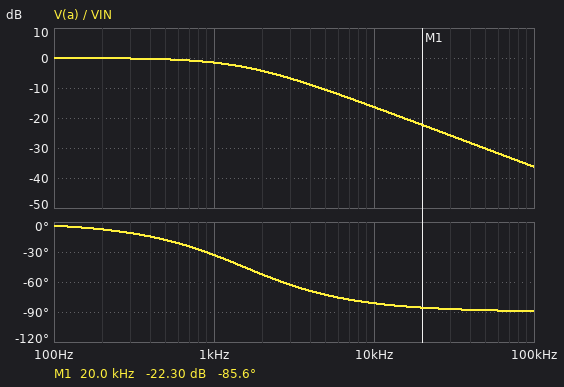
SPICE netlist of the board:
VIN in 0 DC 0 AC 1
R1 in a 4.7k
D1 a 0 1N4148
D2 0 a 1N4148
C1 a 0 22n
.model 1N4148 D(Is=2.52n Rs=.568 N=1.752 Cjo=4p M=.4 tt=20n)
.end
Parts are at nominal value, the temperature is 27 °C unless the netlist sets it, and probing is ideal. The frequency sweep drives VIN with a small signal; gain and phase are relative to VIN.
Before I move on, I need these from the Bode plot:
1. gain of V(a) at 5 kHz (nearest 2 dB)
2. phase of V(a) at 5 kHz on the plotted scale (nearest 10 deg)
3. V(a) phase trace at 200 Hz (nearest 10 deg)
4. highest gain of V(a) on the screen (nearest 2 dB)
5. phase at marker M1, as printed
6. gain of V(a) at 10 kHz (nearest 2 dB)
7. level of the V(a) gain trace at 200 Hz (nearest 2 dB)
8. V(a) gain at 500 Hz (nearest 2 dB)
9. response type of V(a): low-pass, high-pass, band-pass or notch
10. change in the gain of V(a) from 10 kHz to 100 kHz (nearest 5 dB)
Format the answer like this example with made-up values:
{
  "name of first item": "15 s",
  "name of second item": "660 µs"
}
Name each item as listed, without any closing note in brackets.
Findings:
{
  "gain of V(a) at 5 kHz": "-10 dB",
  "phase of V(a) at 5 kHz on the plotted scale": "-70 deg",
  "V(a) phase trace at 200 Hz": "-10 deg",
  "highest gain of V(a) on the screen": "0 dB",
  "phase at marker M1, as printed": "-85.6 deg",
  "gain of V(a) at 10 kHz": "-16 dB",
  "level of the V(a) gain trace at 200 Hz": "0 dB",
  "V(a) gain at 500 Hz": "0 dB",
  "response type of V(a): low-pass, high-pass, band-pass or notch": "low-pass",
  "change in the gain of V(a) from 10 kHz to 100 kHz": "-20 dB"
}
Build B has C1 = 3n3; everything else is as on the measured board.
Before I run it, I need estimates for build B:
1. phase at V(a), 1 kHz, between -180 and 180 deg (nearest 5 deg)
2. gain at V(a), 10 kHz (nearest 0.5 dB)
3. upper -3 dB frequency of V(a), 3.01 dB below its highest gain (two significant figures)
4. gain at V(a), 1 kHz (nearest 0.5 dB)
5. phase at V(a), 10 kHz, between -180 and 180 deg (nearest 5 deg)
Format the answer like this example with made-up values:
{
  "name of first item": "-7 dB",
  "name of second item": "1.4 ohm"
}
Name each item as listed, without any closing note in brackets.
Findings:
{
  "phase at V(a), 1 kHz, between -180 and 180 deg": "-5 deg",
  "gain at V(a), 10 kHz": "-3.0 dB",
  "upper -3 dB frequency of V(a), 3.01 dB below its highest gain": "10 kHz",
  "gain at V(a), 1 kHz": "0 dB",
  "phase at V(a), 10 kHz, between -180 and 180 deg": "-45 deg"
}
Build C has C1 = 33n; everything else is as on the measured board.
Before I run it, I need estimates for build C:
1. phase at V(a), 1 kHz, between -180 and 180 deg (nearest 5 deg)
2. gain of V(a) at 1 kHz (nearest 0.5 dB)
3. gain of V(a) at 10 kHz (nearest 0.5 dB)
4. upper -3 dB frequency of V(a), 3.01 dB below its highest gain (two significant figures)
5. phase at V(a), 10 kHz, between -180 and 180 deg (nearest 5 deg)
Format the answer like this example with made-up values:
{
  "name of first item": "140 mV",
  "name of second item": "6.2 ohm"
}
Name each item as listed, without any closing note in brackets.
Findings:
{
  "phase at V(a), 1 kHz, between -180 and 180 deg": "-45 deg",
  "gain of V(a) at 1 kHz": "-3.0 dB",
  "gain of V(a) at 10 kHz": "-20.0 dB",
  "upper -3 dB frequency of V(a), 3.01 dB below its highest gain": "1.0 kHz",
  "phase at V(a), 10 kHz, between -180 and 180 deg": "-85 deg"
}
